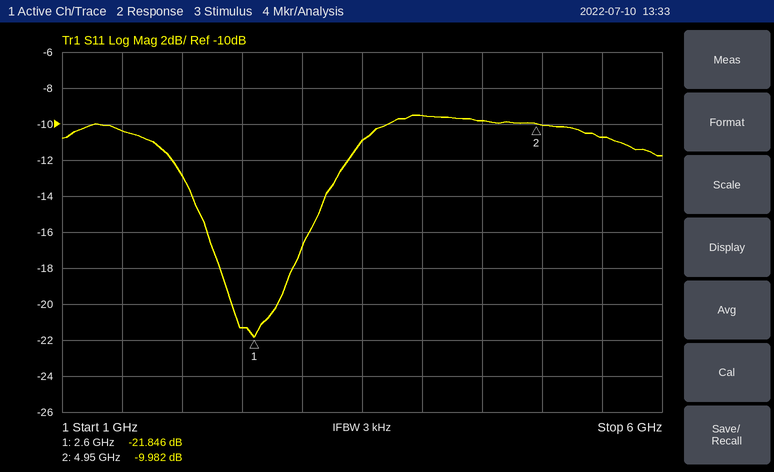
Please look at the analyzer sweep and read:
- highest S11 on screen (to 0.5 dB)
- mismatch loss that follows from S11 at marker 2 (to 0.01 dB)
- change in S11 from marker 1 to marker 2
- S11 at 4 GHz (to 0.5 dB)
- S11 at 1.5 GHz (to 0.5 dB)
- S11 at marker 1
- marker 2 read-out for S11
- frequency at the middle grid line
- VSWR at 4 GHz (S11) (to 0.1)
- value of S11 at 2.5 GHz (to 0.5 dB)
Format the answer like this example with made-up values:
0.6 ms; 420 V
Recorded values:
-9.5 dB; 0.46 dB; 11.864 dB; -9.5 dB; -10.5 dB; -21.846 dB; -9.982 dB; 3.5 GHz; 2.0; -21.5 dB
